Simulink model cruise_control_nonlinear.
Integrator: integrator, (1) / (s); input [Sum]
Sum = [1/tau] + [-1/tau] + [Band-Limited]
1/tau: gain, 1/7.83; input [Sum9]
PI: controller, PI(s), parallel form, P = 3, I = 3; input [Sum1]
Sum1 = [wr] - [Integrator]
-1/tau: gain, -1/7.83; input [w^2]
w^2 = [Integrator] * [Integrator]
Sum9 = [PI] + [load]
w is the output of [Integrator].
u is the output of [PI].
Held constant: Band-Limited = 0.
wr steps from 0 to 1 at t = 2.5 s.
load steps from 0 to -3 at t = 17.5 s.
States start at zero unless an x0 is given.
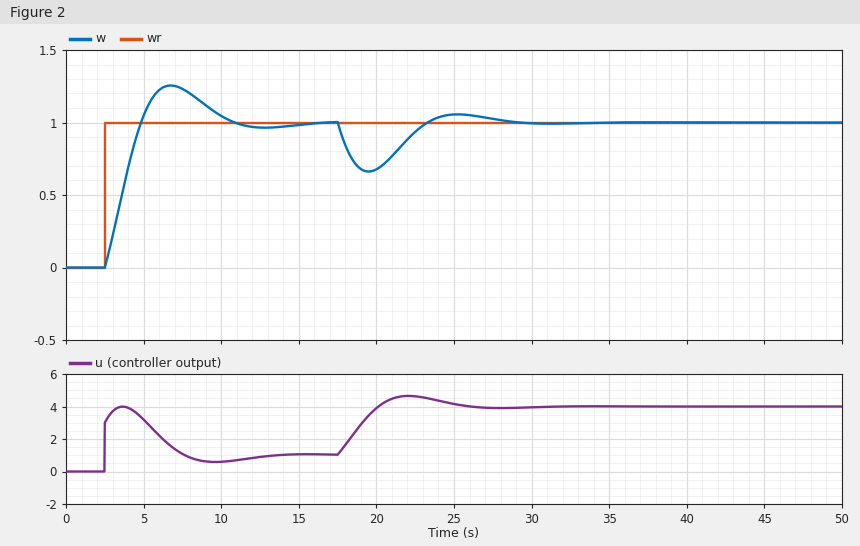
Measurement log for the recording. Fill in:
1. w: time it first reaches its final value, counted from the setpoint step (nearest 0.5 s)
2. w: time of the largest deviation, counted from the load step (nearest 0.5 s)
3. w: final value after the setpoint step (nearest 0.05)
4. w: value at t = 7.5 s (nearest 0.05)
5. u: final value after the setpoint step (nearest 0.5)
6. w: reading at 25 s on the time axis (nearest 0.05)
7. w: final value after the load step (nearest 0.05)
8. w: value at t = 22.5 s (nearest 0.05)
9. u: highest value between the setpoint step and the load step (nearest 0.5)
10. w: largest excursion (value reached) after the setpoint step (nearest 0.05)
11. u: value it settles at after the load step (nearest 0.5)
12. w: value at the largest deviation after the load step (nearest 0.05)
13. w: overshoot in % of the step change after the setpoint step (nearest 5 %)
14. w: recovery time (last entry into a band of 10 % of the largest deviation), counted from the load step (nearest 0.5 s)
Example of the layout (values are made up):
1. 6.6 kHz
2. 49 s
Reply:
1. 2.5 s
2. 2.0 s
3. 1.00
4. 1.25
5. 1.0
6. 1.05
7. 1.00
8. 0.95
9. 4.0
10. 1.25
11. 4.0
12. 0.65
13. 25 %
14. 9.5 s
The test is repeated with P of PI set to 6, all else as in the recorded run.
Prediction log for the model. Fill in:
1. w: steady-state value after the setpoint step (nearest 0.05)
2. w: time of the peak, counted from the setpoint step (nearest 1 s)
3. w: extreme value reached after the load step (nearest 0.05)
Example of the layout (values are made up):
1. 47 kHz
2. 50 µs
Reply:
1. 1.00
2. 4 s
3. 0.75
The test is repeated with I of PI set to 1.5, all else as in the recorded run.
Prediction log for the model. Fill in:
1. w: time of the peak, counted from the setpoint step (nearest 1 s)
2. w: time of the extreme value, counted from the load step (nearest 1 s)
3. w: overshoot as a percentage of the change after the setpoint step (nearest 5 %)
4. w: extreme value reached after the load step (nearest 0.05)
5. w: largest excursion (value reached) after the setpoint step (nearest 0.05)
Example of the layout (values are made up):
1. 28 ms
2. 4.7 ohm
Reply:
1. 6 s
2. 3 s
3. 15 %
4. 0.60
5. 1.15
